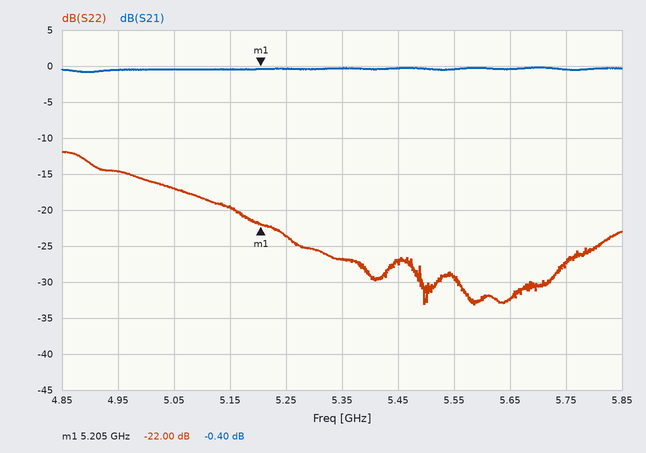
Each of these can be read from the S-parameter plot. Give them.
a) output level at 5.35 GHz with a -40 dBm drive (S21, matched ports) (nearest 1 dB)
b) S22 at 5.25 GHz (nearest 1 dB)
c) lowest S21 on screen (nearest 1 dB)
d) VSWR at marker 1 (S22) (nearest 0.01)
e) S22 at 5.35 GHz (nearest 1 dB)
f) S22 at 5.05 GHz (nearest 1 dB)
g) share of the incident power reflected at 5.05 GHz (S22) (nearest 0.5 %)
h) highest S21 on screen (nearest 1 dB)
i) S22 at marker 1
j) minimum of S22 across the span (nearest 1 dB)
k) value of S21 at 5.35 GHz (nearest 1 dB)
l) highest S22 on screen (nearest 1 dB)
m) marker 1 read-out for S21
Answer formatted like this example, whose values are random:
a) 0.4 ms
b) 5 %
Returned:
a) -40 dBm
b) -24 dB
c) -1 dB
d) 1.17
e) -27 dB
f) -17 dB
g) 2.0 %
h) 0 dB
i) -22.00 dB
j) -33 dB
k) 0 dB
l) -12 dB
m) -0.40 dB
